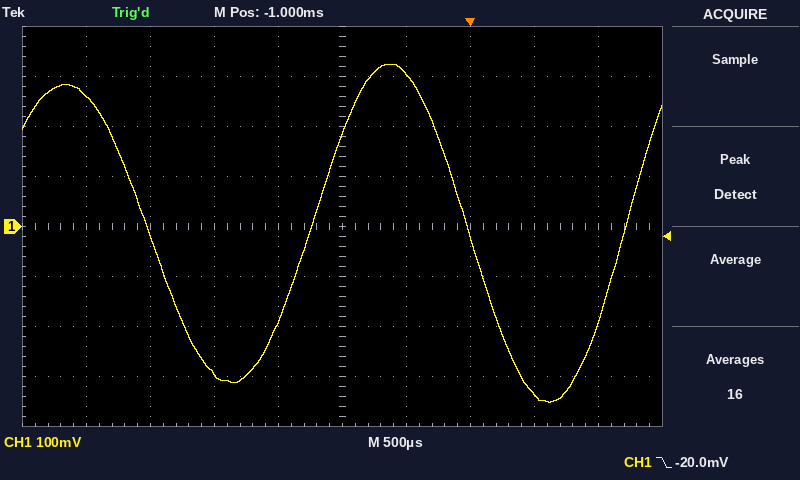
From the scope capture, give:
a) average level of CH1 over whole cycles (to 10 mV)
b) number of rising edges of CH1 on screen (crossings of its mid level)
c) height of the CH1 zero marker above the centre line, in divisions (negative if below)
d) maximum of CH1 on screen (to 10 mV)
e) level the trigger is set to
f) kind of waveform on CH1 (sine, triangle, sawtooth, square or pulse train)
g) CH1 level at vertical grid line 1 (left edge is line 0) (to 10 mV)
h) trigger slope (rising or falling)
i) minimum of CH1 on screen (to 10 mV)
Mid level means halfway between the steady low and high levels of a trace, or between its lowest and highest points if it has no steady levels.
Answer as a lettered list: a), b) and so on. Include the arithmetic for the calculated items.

a) (320 mV + (-350 mV)) / 2 ≈ -15.0 mV, so -10 mV to the nearest 10 mV
b) 2
c) 0.0 div
d) 320 mV
e) -20.0 mV
f) sine
g) 260 mV
h) falling
i) -350 mV
